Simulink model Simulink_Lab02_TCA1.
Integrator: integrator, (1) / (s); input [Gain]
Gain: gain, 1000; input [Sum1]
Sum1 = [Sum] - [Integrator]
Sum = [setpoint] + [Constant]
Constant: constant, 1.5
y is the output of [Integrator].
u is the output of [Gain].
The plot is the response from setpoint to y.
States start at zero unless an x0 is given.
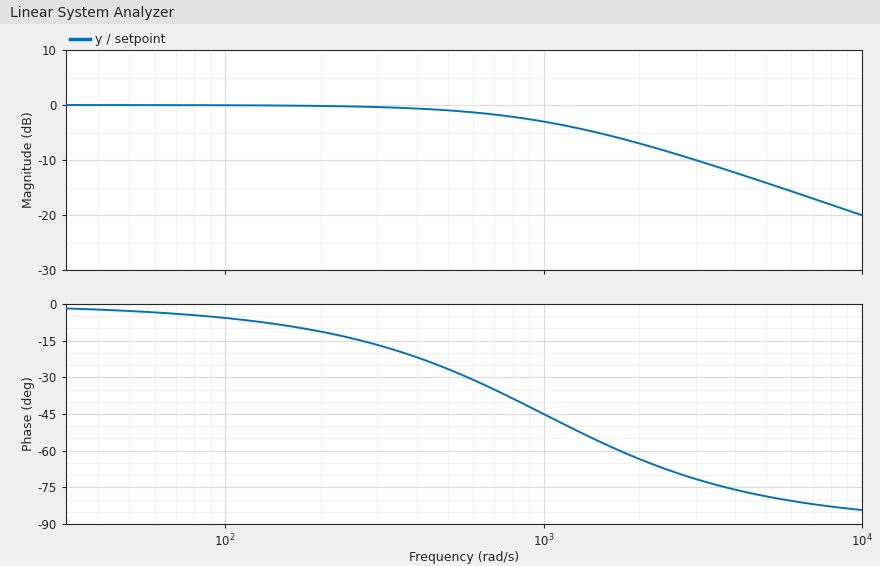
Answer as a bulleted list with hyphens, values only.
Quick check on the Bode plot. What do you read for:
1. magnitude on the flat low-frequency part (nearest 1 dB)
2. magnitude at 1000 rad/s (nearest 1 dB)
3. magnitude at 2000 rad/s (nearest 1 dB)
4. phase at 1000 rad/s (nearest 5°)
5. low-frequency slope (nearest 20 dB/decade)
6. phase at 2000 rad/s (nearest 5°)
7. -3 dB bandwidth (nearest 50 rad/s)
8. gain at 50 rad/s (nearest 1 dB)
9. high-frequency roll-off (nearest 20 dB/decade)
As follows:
- 0 dB
- -3 dB
- -7 dB
- -45°
- 0 dB/decade
- -65°
- 1000 rad/s
- 0 dB
- -20 dB/decade
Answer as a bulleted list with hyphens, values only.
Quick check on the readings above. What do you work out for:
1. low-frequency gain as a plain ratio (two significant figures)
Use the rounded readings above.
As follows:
- 1.0
